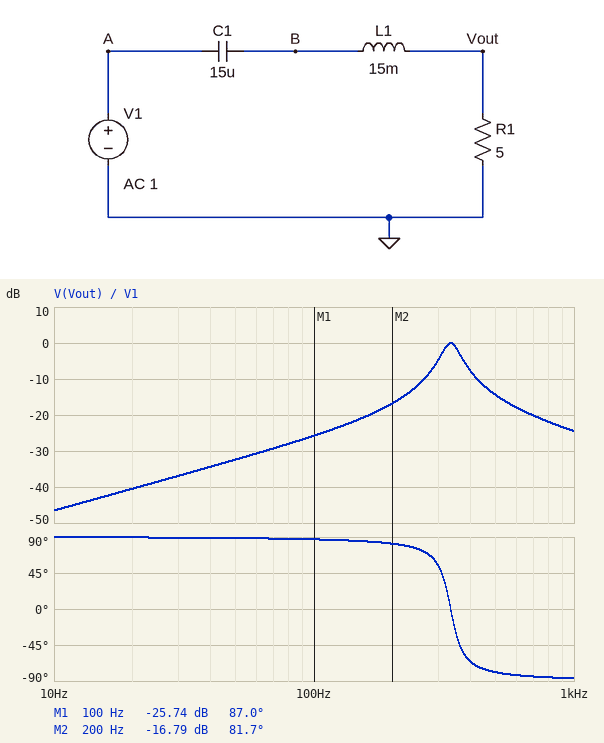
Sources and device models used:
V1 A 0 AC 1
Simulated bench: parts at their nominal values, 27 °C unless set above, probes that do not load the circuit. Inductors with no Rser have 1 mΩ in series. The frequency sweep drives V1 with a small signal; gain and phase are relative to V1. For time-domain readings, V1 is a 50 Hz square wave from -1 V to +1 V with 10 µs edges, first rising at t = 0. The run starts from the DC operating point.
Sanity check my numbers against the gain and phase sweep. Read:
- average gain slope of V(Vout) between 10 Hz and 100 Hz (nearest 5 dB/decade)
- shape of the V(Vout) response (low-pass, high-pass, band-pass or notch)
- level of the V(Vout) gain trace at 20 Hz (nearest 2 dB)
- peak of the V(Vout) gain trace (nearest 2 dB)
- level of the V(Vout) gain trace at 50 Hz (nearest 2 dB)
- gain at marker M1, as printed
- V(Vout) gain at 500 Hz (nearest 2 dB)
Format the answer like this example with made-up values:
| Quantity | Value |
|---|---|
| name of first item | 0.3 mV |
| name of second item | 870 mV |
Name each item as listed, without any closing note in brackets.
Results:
| Quantity | Value |
|---|---|
| average gain slope of V(Vout) between 10 Hz and 100 Hz | 20 dB/decade |
| shape of the V(Vout) response | band-pass |
| level of the V(Vout) gain trace at 20 Hz | -40 dB |
| peak of the V(Vout) gain trace | 0 dB |
| level of the V(Vout) gain trace at 50 Hz | -32 dB |
| gain at marker M1, as printed | -25.74 dB |
| V(Vout) gain at 500 Hz | -14 dB |
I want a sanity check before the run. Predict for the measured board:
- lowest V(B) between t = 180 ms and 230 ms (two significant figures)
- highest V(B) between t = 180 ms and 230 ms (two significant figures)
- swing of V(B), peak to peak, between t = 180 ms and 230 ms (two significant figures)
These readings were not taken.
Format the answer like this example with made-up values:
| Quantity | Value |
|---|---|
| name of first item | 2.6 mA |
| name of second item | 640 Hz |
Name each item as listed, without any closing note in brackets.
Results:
| Quantity | Value |
|---|---|
| lowest V(B) between t = 180 ms and 230 ms | -2.2 V |
| highest V(B) between t = 180 ms and 230 ms | 2.2 V |
| swing of V(B), peak to peak, between t = 180 ms and 230 ms | 4.3 V |
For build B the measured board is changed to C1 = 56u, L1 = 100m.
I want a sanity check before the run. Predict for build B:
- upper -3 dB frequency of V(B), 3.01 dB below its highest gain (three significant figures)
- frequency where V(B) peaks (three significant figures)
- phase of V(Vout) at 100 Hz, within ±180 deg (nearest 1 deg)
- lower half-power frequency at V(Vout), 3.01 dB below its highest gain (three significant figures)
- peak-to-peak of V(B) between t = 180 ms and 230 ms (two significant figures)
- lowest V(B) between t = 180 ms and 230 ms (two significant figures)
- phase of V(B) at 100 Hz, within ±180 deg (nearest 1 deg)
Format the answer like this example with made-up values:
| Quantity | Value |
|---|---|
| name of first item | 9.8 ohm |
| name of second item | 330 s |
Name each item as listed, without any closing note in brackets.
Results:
| Quantity | Value |
|---|---|
| upper -3 dB frequency of V(B), 3.01 dB below its highest gain | 71.9 Hz |
| frequency where V(B) peaks | 67.5 Hz |
| phase of V(Vout) at 100 Hz, within ±180 deg | -82 deg |
| lower half-power frequency at V(Vout), 3.01 dB below its highest gain | 63.4 Hz |
| peak-to-peak of V(B) between t = 180 ms and 230 ms | 3.8 V |
| lowest V(B) between t = 180 ms and 230 ms | -1.9 V |
| phase of V(B) at 100 Hz, within ±180 deg | 4 deg |
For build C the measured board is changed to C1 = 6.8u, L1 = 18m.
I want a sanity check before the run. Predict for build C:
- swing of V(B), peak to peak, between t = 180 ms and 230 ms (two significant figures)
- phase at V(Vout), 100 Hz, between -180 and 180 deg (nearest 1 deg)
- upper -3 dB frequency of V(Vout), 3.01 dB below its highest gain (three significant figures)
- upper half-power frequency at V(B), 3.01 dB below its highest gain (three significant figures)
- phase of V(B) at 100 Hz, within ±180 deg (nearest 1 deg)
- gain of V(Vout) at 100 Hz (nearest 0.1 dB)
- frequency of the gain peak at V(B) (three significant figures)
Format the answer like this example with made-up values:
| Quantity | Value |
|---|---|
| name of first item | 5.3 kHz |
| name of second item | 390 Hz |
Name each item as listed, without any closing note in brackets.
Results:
| Quantity | Value |
|---|---|
| swing of V(B), peak to peak, between t = 180 ms and 230 ms | 5.3 V |
| phase at V(Vout), 100 Hz, between -180 and 180 deg | 89 deg |
| upper -3 dB frequency of V(Vout), 3.01 dB below its highest gain | 478 Hz |
| upper half-power frequency at V(B), 3.01 dB below its highest gain | 480 Hz |
| phase of V(B) at 100 Hz, within ±180 deg | 155 deg |
| gain of V(Vout) at 100 Hz | -33.0 dB |
| frequency of the gain peak at V(B) | 456 Hz |
